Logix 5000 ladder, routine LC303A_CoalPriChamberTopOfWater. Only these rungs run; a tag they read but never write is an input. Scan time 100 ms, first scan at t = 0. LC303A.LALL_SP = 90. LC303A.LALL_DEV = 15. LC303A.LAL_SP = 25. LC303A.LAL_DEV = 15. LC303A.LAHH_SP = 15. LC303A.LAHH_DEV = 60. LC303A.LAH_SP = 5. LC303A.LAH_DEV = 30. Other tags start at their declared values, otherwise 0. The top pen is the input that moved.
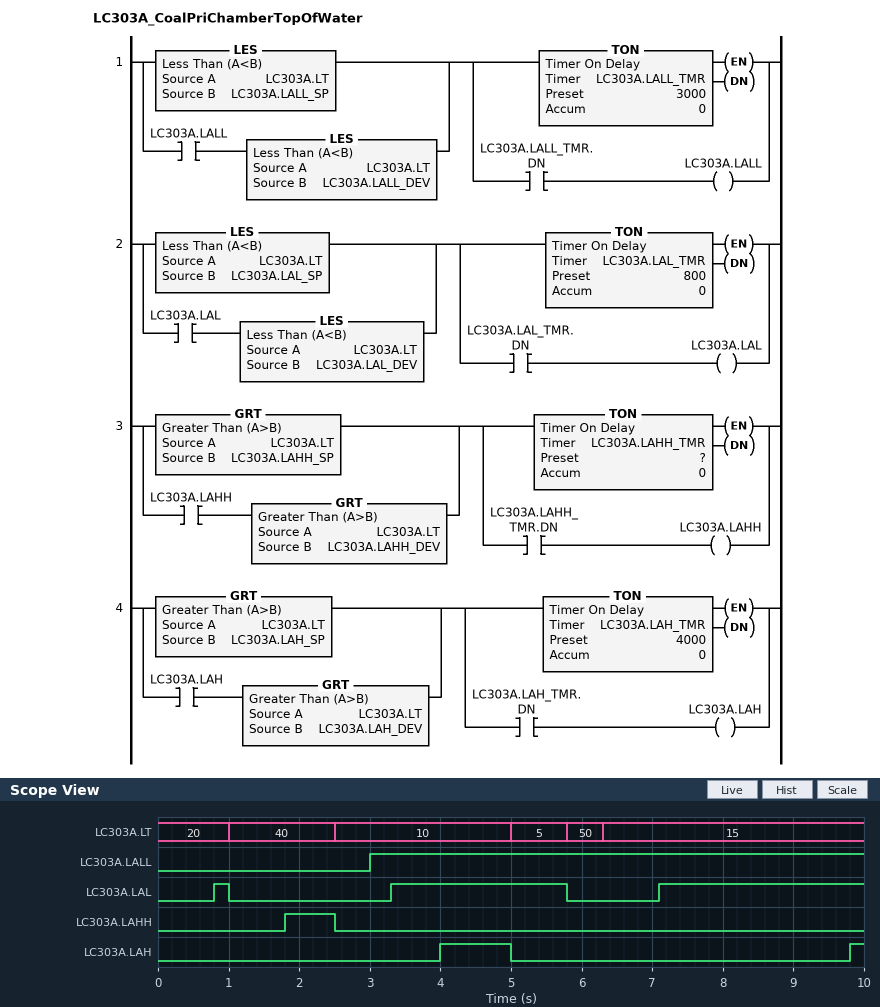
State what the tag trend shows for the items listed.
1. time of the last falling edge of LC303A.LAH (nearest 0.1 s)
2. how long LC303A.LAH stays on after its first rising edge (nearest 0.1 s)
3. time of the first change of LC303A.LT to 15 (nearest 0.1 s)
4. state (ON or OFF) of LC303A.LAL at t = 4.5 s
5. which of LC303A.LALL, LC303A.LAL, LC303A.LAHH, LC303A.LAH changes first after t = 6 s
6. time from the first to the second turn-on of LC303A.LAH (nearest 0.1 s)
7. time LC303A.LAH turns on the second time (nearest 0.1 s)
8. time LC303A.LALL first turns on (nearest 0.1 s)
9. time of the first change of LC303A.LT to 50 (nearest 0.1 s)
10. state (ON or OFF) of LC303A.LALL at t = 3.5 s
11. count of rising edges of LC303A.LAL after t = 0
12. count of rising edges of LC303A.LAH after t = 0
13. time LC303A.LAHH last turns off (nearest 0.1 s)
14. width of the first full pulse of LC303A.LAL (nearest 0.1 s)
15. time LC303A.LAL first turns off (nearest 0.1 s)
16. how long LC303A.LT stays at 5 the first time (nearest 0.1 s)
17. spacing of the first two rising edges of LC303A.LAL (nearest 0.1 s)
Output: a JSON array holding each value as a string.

["5.0 s", "1.0 s", "6.3 s", "ON", "LC303A.LAL", "5.8 s", "9.8 s", "3.0 s", "5.8 s", "ON", "3", "2", "2.5 s", "0.2 s", "1.0 s", "0.8 s", "2.5 s"]
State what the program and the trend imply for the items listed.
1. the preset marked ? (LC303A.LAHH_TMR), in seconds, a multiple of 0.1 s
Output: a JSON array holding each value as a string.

["1.8 s"]
